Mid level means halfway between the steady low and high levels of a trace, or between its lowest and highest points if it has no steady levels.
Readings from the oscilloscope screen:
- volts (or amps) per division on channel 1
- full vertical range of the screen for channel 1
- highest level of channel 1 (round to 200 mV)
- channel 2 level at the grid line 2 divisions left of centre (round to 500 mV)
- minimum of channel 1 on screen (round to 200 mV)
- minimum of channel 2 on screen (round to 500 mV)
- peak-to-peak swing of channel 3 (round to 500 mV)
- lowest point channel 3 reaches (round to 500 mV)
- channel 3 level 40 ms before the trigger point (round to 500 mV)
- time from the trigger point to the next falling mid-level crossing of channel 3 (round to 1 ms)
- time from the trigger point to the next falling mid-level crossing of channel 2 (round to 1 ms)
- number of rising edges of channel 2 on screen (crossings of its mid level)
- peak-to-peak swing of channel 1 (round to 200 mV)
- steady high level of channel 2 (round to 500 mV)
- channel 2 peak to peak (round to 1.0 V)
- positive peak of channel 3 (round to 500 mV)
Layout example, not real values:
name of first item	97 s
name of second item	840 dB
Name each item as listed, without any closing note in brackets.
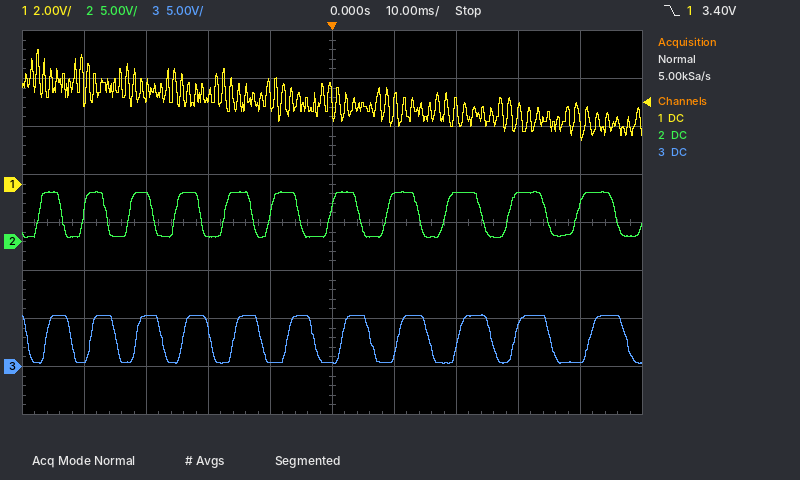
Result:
volts (or amps) per division on channel 1	2 V
full vertical range of the screen for channel 1	16 V
highest level of channel 1	5.6 V
channel 2 level at the grid line 2 divisions left of centre	500 mV
minimum of channel 1 on screen	1.8 V
minimum of channel 2 on screen	500 mV
peak-to-peak swing of channel 3	5.0 V
lowest point channel 3 reaches	500 mV
channel 3 level 40 ms before the trigger point	500 mV
time from the trigger point to the next falling mid-level crossing of channel 3	6 ms
time from the trigger point to the next falling mid-level crossing of channel 2	4 ms
number of rising edges of channel 2 on screen	11
peak-to-peak swing of channel 1	3.8 V
steady high level of channel 2	5.0 V
channel 2 peak to peak	5.0 V
positive peak of channel 3	5.5 V
